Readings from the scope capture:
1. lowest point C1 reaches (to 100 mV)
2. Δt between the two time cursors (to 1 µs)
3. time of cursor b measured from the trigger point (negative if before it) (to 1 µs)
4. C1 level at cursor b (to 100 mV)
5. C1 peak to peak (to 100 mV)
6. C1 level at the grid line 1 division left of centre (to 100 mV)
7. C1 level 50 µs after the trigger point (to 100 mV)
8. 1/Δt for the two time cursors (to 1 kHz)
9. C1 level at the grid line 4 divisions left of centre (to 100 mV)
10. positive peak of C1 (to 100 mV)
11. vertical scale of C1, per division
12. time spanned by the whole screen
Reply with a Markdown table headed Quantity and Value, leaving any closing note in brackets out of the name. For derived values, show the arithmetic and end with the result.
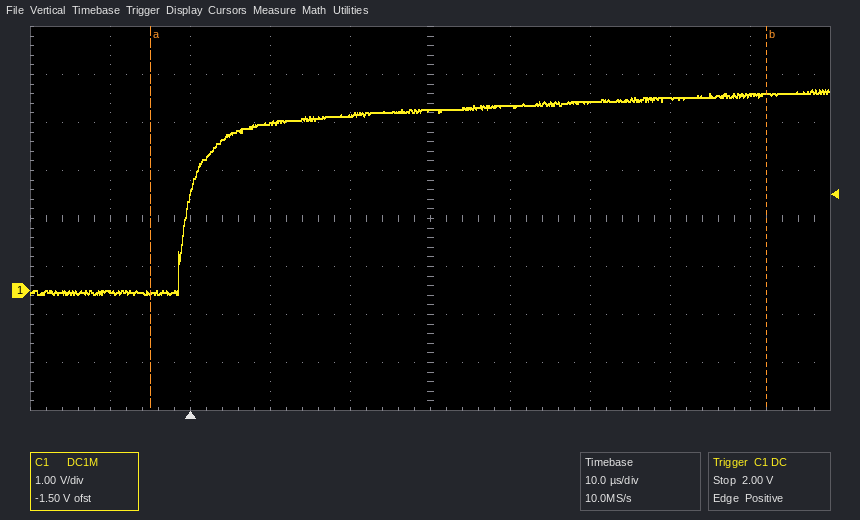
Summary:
| Quantity | Value |
|---|---|
| lowest point C1 reaches | -100 mV |
| Δt between the two time cursors | 77 µs |
| time of cursor b measured from the trigger point (negative if before it) | +72 µs |
| C1 level at cursor b | 4.1 V |
| C1 peak to peak | 4.2 V − (-100 mV) = 4.3 V |
| C1 level at the grid line 1 division left of centre | 3.6 V |
| C1 level 50 µs after the trigger point | 3.9 V |
| 1/Δt for the two time cursors | 1 / 77 µs ≈ 13 kHz |
| C1 level at the grid line 4 divisions left of centre | 0.0 V |
| positive peak of C1 | 4.2 V |
| vertical scale of C1, per division | 1 V |
| time spanned by the whole screen | 100 µs |
